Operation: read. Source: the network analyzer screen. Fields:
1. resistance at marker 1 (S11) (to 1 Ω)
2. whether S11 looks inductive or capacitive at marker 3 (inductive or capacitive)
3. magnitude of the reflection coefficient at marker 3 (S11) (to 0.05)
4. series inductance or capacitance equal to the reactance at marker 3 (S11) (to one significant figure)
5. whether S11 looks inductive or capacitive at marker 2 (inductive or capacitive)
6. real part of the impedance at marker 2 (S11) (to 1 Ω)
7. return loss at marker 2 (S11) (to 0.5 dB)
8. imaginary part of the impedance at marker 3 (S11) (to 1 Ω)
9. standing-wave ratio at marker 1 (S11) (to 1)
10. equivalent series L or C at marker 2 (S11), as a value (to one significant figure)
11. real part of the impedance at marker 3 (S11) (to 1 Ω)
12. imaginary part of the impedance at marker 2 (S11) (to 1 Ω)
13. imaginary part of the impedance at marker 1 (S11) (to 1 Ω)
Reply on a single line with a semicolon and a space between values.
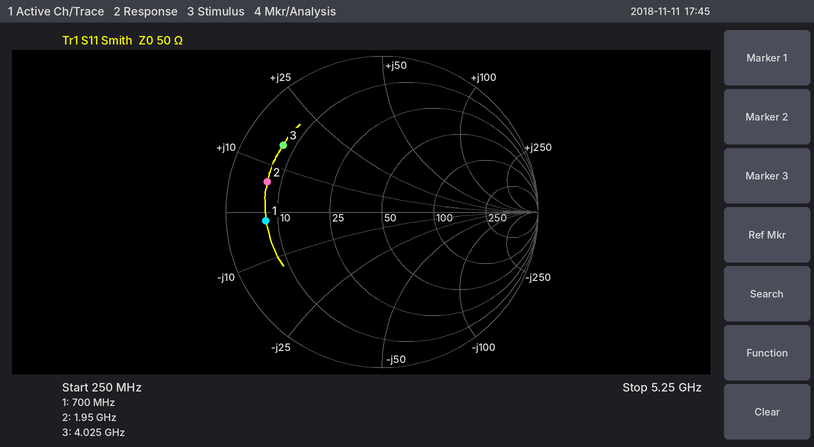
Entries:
7 Ω; inductive; 0.75; 600 pH; inductive; 7 Ω; 2.5 dB; +15 Ω; 7; 500 pH; 7 Ω; +6 Ω; -2 Ω
